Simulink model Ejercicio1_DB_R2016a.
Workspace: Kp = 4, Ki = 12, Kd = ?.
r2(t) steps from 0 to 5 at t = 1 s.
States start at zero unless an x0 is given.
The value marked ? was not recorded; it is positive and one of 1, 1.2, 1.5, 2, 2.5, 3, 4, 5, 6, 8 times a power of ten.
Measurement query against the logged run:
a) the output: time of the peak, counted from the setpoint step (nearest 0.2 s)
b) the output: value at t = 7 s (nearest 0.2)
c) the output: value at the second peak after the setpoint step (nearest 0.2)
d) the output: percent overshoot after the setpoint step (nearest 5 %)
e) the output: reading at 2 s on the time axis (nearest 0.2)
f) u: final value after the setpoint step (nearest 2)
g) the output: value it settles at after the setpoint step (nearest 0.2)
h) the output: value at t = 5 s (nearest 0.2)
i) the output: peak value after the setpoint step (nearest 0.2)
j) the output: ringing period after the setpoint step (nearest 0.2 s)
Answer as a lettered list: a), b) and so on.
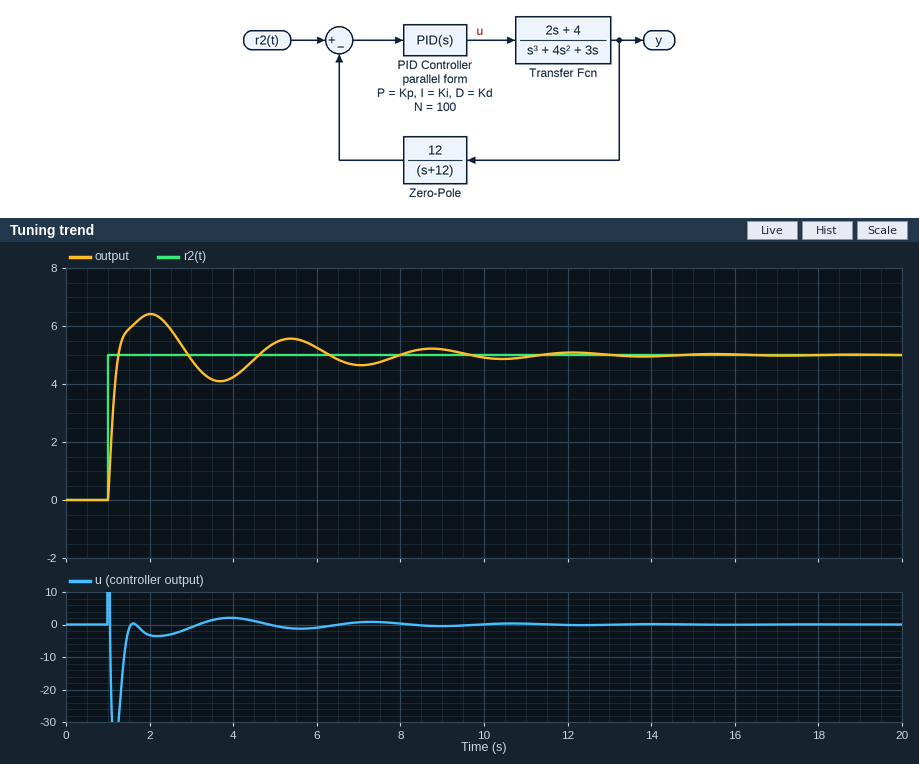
a) 1.0 s
b) 4.6
c) 5.6
d) 30 %
e) 6.4
f) 0
g) 5.0
h) 5.4
i) 6.4
j) 3.4 s
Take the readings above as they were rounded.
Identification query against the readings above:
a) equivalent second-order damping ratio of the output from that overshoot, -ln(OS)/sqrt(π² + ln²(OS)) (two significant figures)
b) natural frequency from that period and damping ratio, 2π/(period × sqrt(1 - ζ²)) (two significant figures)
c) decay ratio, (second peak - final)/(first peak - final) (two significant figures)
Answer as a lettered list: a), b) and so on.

a) 0.36
b) 2.0 rad/s
c) 0.43
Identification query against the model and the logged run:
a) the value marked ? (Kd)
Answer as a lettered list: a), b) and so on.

a) 3
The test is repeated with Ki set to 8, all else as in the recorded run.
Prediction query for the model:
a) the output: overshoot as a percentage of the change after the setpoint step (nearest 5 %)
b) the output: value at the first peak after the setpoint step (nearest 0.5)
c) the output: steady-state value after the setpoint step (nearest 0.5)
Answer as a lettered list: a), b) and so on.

a) 20 %
b) 6.0
c) 5.0
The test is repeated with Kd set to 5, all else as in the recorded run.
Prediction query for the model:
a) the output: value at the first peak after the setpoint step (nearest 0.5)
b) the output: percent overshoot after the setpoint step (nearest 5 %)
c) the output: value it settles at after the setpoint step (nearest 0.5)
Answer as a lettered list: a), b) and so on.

a) 6.0
b) 20 %
c) 5.0
